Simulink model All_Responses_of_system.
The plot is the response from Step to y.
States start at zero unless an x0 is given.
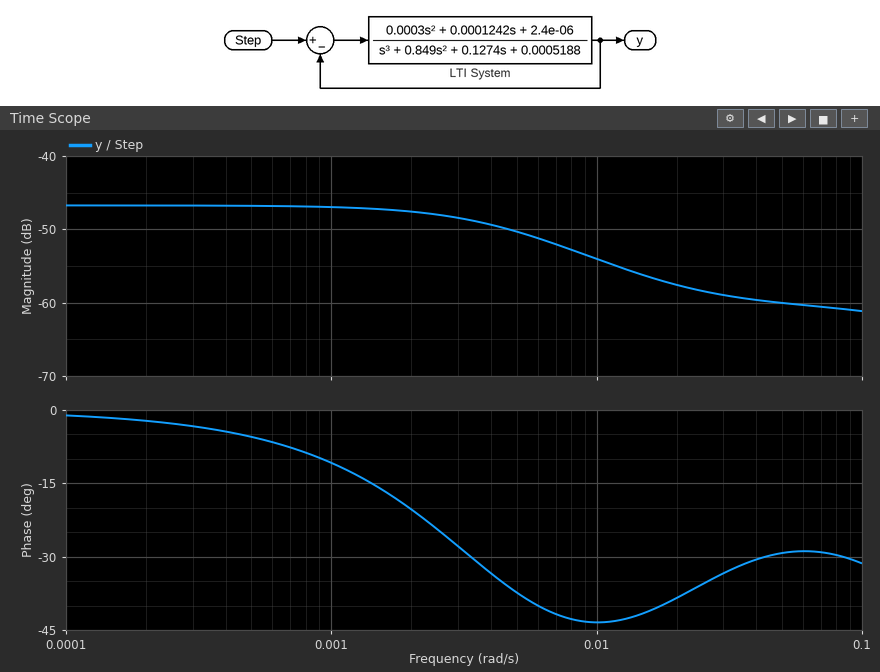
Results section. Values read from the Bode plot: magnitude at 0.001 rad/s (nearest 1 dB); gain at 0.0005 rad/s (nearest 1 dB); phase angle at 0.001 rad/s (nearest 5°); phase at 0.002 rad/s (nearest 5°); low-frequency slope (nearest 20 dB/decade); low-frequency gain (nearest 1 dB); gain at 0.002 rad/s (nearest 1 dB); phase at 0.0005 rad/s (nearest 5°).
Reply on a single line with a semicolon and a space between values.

-47 dB; -47 dB; -10°; -20°; 0 dB/decade; -47 dB; -48 dB; -5°
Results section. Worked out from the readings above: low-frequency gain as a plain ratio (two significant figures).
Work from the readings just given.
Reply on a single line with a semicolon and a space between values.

0.0045
